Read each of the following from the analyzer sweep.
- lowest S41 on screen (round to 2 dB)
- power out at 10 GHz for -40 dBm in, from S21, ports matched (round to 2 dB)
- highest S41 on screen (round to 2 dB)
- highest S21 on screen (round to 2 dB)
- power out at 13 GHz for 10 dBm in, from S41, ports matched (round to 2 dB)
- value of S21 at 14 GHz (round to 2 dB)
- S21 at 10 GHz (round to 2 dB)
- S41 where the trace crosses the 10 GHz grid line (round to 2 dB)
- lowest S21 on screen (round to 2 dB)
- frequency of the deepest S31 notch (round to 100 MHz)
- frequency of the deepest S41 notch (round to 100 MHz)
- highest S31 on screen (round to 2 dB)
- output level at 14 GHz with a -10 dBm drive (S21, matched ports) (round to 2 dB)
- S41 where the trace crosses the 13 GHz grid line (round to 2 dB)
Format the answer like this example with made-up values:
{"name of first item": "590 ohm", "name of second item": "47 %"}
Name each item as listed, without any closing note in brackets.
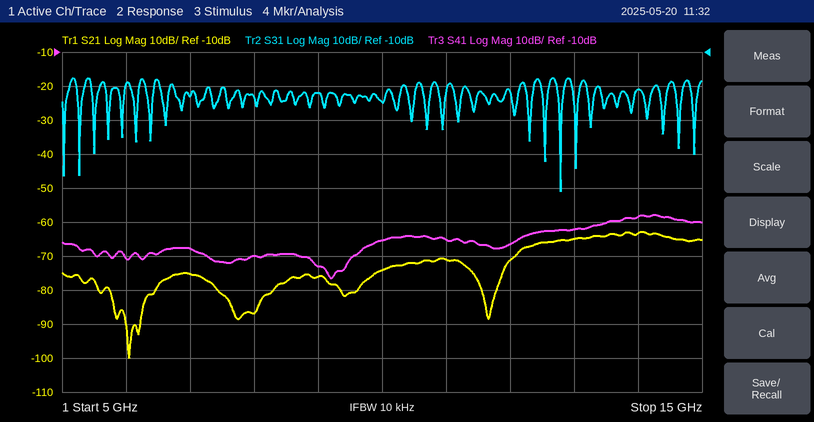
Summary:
{"lowest S41 on screen": "-76 dB", "power out at 10 GHz for -40 dBm in, from S21, ports matched": "-114 dBm", "highest S41 on screen": "-58 dB", "highest S21 on screen": "-62 dB", "power out at 13 GHz for 10 dBm in, from S41, ports matched": "-52 dBm", "value of S21 at 14 GHz": "-64 dB", "S21 at 10 GHz": "-74 dB", "S41 where the trace crosses the 10 GHz grid line": "-66 dB", "lowest S21 on screen": "-100 dB", "frequency of the deepest S31 notch": "12.8 GHz", "frequency of the deepest S41 notch": "9.2 GHz", "highest S31 on screen": "-18 dB", "output level at 14 GHz with a -10 dBm drive (S21, matched ports)": "-74 dBm", "S41 where the trace crosses the 13 GHz grid line": "-62 dB"}
